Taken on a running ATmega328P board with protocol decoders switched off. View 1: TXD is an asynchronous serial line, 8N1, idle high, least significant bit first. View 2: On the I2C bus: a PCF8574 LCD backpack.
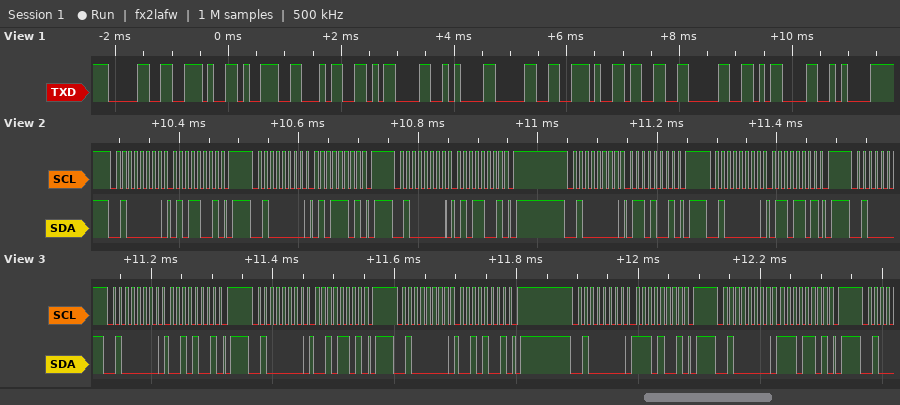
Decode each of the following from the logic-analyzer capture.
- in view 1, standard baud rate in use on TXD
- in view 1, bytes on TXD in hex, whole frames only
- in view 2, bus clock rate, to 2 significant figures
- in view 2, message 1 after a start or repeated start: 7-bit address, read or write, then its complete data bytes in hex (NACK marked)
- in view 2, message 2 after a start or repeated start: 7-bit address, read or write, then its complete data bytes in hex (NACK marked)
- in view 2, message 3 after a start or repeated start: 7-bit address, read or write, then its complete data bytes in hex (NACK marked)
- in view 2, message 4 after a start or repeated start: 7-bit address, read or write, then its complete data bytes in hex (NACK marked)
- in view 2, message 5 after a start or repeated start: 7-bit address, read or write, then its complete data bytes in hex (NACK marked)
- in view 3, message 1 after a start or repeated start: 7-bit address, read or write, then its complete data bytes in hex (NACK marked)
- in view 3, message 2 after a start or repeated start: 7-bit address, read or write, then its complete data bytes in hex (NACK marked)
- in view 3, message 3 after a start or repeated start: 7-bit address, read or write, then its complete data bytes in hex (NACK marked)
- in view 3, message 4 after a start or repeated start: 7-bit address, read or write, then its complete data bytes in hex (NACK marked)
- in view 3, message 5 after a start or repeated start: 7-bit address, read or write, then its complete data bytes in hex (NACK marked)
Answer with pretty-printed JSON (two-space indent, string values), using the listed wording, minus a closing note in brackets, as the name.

{
  "in view 1, standard baud rate in use on TXD": "9600 baud",
  "in view 1, bytes on TXD in hex, whole frames only": "0x30 0x2E 0x39 0x34 0x0D 0x0A 0x30 0x2E 0x33 0x30 0x0D 0x0A",
  "in view 2, bus clock rate, to 2 significant figures": "100 kHz",
  "in view 2, message 1 after a start or repeated start: 7-bit address, read or write, then its complete data bytes in hex": "0x20 write: 59",
  "in view 2, message 2 after a start or repeated start: 7-bit address, read or write, then its complete data bytes in hex": "0x20 write: 5D",
  "in view 2, message 3 after a start or repeated start: 7-bit address, read or write, then its complete data bytes in hex": "0x20 write: 59",
  "in view 2, message 4 after a start or repeated start: 7-bit address, read or write, then its complete data bytes in hex": "0x20 write: 69",
  "in view 2, message 5 after a start or repeated start: 7-bit address, read or write, then its complete data bytes in hex": "0x20 write: 6D",
  "in view 3, message 1 after a start or repeated start: 7-bit address, read or write, then its complete data bytes in hex": "0x20 write: 29",
  "in view 3, message 2 after a start or repeated start: 7-bit address, read or write, then its complete data bytes in hex": "0x20 write: 2D",
  "in view 3, message 3 after a start or repeated start: 7-bit address, read or write, then its complete data bytes in hex": "0x20 write: 29",
  "in view 3, message 4 after a start or repeated start: 7-bit address, read or write, then its complete data bytes in hex": "0x20 write: E9",
  "in view 3, message 5 after a start or repeated start: 7-bit address, read or write, then its complete data bytes in hex": "0x20 write: ED"
}
